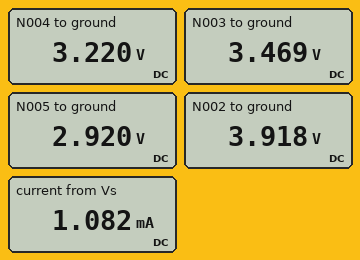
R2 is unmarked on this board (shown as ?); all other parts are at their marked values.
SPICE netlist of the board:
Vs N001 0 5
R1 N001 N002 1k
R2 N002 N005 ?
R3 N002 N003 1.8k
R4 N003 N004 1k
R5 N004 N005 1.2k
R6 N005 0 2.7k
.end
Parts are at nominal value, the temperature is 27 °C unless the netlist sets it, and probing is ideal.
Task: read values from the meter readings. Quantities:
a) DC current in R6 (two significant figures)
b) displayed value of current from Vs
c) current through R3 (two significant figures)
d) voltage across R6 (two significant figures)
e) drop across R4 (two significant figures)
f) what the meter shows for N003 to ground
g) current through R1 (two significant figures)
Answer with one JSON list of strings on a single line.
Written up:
["1.1 mA", "1.082 mA", "250 µA", "2.9 V", "250 mV", "3.469 V", "1.1 mA"]
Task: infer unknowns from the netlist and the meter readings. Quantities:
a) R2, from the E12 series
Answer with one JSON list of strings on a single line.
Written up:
["1.2 kΩ"]
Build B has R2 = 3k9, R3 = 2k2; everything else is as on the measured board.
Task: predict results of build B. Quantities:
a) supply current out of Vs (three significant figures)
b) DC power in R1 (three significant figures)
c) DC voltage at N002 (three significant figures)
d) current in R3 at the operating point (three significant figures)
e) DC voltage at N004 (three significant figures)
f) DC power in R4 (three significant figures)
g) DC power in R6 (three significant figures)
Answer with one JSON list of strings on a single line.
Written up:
["867 µA", "752 µW", "4.13 V", "407 µA", "2.83 V", "166 µW", "2.03 mW"]
